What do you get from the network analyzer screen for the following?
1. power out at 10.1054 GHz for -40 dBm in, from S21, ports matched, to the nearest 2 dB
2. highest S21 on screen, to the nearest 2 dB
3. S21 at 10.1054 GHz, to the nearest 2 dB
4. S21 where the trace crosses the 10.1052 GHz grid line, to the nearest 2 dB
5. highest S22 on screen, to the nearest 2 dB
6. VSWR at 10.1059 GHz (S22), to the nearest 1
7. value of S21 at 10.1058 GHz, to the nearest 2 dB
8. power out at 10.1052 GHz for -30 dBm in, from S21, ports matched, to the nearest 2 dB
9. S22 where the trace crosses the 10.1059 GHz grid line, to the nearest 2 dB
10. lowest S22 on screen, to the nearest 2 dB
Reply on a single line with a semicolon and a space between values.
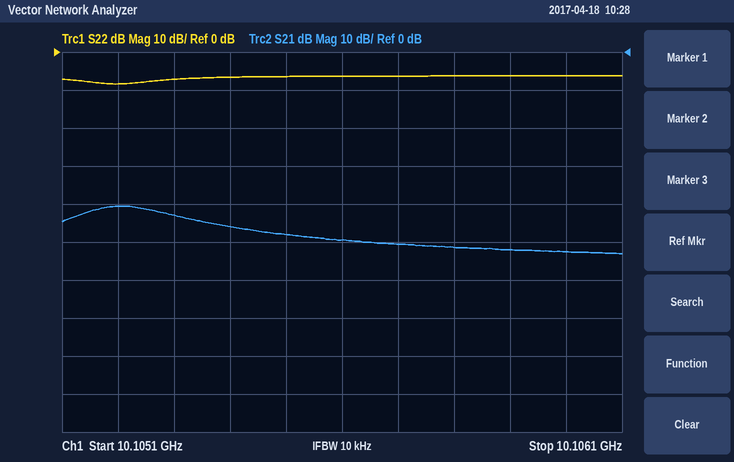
-86 dBm; -40 dB; -46 dB; -40 dB; -6 dB; 3; -52 dB; -70 dBm; -6 dB; -8 dB
